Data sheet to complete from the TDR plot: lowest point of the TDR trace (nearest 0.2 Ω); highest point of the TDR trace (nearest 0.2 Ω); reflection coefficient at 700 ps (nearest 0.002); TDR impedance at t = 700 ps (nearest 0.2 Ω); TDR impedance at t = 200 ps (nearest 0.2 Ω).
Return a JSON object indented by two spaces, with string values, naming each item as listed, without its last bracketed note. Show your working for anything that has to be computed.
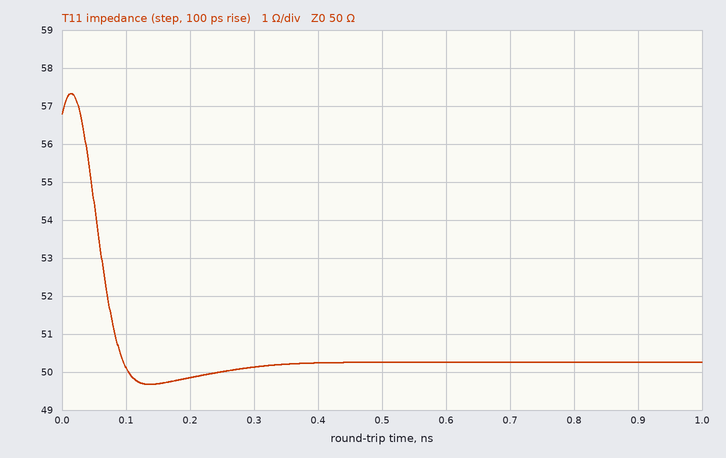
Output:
{
  "lowest point of the TDR trace": "49.6 Ω",
  "highest point of the TDR trace": "57.4 Ω",
  "reflection coefficient at 700 ps": "(50.2 − 50)/(50.2 + 50) ≈ +0.002",
  "TDR impedance at t = 700 ps": "50.2 Ω",
  "TDR impedance at t = 200 ps": "49.8 Ω"
}
